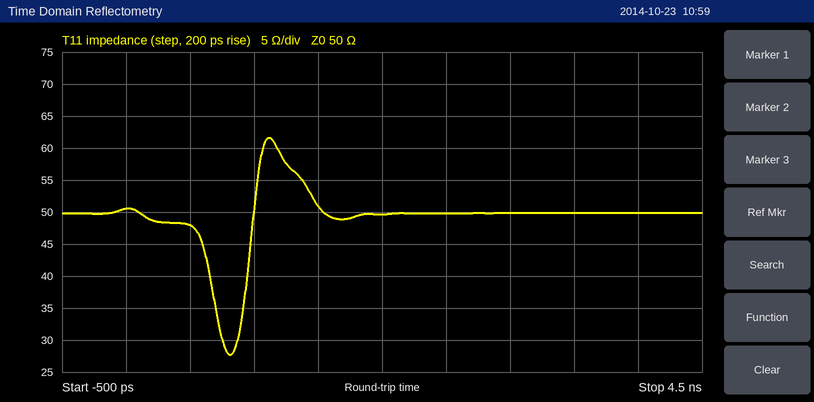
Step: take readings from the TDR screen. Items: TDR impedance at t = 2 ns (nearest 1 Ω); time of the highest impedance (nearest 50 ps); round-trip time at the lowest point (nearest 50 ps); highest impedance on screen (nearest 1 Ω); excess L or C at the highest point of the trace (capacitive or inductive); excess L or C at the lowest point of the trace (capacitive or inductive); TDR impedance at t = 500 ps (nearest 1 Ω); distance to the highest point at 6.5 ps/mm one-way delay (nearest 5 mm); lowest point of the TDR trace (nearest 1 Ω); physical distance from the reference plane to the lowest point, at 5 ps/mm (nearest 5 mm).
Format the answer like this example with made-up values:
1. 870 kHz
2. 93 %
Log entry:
1. 50 Ω
2. 1.10 ns
3. 800 ps
4. 62 Ω
5. inductive
6. capacitive
7. 48 Ω
8. 85 mm
9. 28 Ω
10. 80 mm
